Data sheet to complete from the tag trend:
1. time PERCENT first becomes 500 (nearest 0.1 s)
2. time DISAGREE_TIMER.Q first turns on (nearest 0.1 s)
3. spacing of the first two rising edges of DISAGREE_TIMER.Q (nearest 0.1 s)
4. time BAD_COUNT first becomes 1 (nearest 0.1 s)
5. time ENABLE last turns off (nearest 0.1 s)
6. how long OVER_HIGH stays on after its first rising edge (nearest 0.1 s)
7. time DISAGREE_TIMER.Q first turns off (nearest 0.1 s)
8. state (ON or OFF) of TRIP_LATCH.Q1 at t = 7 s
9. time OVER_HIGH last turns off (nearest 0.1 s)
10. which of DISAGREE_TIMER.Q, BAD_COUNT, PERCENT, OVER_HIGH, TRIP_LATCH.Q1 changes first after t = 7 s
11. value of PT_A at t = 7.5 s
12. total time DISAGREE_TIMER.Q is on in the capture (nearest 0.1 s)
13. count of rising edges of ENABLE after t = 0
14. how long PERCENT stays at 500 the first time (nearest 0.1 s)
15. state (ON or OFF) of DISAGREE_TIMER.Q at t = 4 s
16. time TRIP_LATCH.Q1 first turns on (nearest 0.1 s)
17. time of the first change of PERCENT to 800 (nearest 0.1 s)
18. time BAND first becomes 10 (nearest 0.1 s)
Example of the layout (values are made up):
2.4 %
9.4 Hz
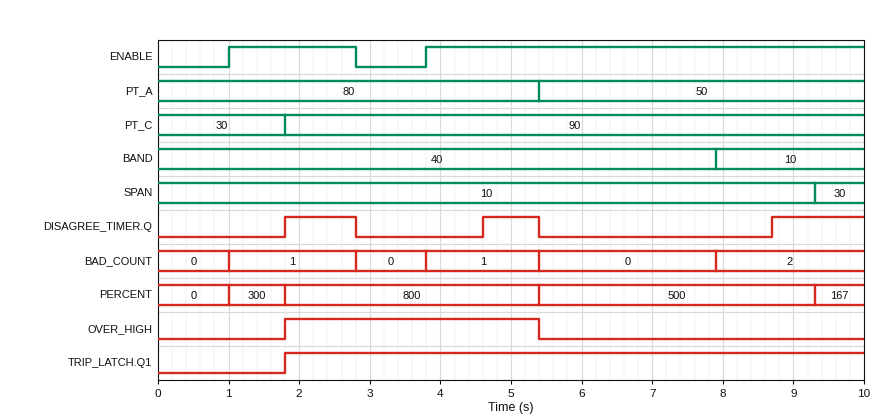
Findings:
5.4 s
1.8 s
2.8 s
1.0 s
2.8 s
3.6 s
2.8 s
ON
5.4 s
BAD_COUNT
50
3.1 s
2
3.9 s
OFF
1.8 s
1.8 s
7.9 s
